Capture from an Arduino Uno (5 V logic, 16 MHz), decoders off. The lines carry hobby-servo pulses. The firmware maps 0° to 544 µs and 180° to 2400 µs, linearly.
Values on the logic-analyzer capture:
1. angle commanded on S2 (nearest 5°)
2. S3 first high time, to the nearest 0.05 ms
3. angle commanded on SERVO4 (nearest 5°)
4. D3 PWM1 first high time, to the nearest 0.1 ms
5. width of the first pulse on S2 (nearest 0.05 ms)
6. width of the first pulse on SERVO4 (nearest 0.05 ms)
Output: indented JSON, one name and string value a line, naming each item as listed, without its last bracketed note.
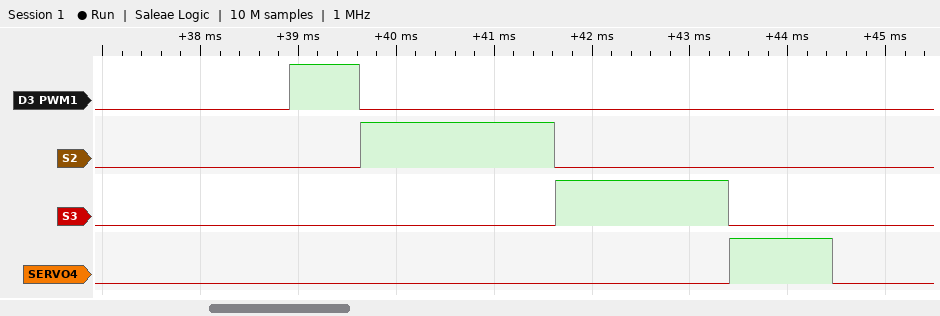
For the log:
{
  "angle commanded on S2": "140°",
  "S3 first high time, to the nearest 0.05 ms": "1.75 ms",
  "angle commanded on SERVO4": "50°",
  "D3 PWM1 first high time, to the nearest 0.1 ms": "0.7 ms",
  "width of the first pulse on S2": "2.00 ms",
  "width of the first pulse on SERVO4": "1.05 ms"
}
